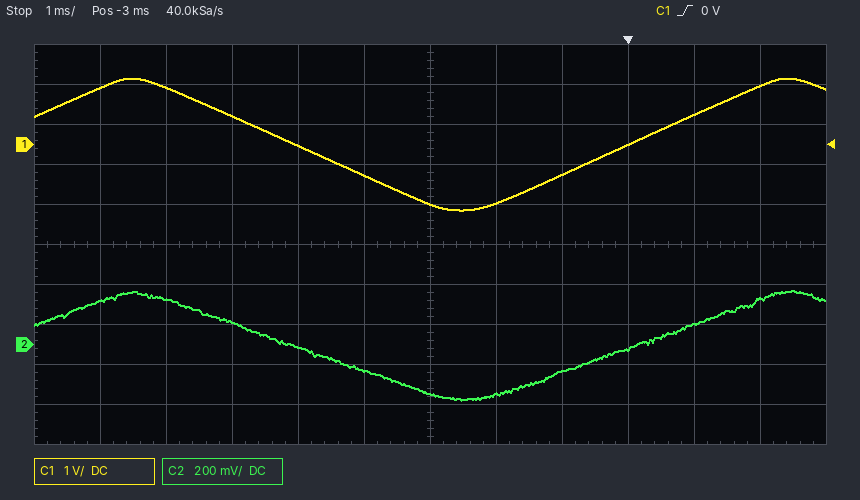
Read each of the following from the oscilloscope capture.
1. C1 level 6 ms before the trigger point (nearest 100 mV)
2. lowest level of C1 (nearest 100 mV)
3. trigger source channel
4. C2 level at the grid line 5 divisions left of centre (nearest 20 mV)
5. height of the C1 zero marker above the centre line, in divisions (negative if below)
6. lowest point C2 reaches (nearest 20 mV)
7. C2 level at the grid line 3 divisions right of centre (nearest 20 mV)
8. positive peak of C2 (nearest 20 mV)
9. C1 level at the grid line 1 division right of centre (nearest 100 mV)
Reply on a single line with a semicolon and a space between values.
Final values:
700 mV; -1.6 V; C1; 220 mV; +2.5 div; -280 mV; -20 mV; 280 mV; -1.5 V
